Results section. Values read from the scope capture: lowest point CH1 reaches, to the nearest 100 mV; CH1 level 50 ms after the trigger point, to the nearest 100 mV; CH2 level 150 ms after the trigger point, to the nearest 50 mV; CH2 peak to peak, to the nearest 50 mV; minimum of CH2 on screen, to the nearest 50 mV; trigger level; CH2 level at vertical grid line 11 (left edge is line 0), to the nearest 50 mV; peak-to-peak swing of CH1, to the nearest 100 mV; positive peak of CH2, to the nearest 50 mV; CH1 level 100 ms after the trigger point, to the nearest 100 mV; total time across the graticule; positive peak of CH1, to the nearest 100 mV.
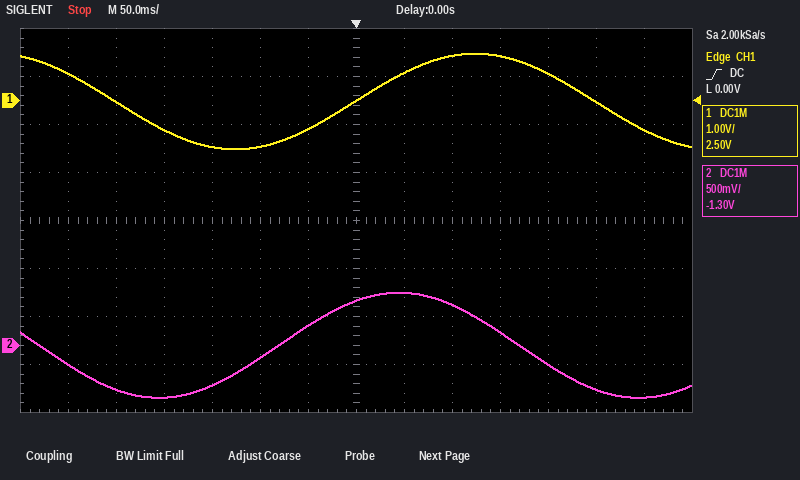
-1.0 V
600 mV
150 mV
1.10 V
-550 mV
0.00 V
-200 mV
2.0 V
550 mV
900 mV
700 ms
1.0 V
